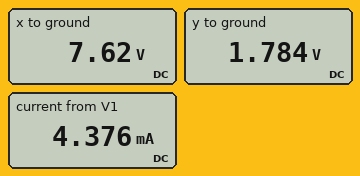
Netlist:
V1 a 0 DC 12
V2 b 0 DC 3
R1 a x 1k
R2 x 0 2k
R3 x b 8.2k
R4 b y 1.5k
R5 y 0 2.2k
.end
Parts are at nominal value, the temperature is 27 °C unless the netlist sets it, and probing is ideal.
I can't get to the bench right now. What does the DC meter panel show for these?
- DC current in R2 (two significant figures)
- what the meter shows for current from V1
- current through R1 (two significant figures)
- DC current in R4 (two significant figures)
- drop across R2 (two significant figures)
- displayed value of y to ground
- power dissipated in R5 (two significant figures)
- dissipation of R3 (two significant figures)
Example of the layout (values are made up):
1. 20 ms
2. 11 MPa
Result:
1. 3.8 mA
2. 4.376 mA
3. 4.4 mA
4. 810 µA
5. 7.6 V
6. 1.784 V
7. 1.4 mW
8. 2.6 mW
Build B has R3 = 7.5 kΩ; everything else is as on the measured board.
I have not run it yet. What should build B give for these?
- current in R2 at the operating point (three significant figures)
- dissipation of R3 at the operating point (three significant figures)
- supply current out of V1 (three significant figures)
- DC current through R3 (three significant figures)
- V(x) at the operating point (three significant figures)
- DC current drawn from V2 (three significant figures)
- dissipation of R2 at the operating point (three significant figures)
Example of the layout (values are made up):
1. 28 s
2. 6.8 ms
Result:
1. 3.80 mA
2. 2.81 mW
3. 4.41 mA
4. 612 µA
5. 7.59 V
6. 199 µA
7. 28.8 mW
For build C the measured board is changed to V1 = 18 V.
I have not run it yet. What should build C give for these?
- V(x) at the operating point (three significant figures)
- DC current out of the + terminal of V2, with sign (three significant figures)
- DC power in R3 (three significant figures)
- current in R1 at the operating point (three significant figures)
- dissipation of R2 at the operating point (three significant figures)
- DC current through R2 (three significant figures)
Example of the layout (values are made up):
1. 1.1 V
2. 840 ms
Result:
1. 11.3 V
2. -204 µA
3. 8.45 mW
4. 6.68 mA
5. 64.1 mW
6. 5.66 mA
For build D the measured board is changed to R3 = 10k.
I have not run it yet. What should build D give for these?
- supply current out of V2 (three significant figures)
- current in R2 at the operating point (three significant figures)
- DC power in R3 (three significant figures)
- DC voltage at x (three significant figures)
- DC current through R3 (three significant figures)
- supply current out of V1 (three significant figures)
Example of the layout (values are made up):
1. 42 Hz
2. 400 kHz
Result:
1. 342 µA
2. 3.84 mA
3. 2.20 mW
4. 7.69 V
5. 469 µA
6. 4.31 mA
